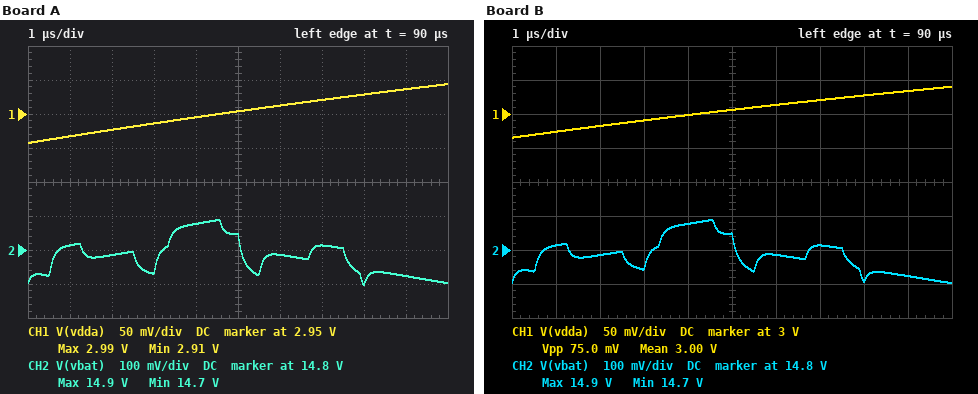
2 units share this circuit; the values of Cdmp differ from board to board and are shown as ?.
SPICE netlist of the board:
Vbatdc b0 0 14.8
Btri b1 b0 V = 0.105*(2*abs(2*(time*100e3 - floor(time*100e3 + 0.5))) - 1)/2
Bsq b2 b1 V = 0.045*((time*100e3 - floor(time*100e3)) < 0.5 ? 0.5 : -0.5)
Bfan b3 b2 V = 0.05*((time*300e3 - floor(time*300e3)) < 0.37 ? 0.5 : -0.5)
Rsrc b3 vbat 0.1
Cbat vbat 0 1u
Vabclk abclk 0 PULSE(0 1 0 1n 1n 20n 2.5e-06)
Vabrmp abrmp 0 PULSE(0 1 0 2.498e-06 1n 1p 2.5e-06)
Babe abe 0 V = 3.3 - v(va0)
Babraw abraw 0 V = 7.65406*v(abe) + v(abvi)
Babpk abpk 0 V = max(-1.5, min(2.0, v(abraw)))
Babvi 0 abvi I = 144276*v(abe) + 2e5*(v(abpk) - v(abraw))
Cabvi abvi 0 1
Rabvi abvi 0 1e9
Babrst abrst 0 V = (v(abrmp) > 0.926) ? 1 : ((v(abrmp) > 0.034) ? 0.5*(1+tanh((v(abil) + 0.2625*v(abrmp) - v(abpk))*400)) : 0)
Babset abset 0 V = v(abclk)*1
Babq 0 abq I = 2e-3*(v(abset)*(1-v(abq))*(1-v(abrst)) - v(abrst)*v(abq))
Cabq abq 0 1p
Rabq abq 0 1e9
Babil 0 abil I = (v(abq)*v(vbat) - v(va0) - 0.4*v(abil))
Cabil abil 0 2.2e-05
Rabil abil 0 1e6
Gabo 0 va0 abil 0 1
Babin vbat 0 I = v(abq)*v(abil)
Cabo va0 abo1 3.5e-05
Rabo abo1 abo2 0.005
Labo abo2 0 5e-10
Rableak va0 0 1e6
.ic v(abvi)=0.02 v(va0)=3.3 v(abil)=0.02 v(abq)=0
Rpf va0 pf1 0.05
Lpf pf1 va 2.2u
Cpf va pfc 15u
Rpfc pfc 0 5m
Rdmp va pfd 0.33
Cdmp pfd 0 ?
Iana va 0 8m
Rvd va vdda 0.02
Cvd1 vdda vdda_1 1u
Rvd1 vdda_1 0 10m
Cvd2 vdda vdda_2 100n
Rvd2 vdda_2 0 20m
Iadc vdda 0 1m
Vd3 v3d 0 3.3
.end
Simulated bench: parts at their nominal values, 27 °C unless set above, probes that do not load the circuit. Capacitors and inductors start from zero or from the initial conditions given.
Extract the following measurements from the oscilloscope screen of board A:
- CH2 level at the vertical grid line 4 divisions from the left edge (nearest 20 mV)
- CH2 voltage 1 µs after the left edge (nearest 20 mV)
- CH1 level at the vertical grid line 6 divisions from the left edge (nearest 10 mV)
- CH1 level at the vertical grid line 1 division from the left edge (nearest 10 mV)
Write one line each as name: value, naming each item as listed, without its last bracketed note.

CH2 level at the vertical grid line 4 divisions from the left edge: 14.88 V
CH2 voltage 1 µs after the left edge: 14.82 V
CH1 level at the vertical grid line 6 divisions from the left edge: 2.96 V
CH1 level at the vertical grid line 1 division from the left edge: 2.92 V
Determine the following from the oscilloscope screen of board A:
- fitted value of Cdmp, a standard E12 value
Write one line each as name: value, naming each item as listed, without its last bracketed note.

fitted value of Cdmp, a standard E12 value: 22 µF
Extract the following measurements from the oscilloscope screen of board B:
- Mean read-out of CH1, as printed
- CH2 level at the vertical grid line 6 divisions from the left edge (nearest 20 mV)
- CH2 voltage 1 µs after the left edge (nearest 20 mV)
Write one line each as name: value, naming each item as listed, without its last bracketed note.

Mean read-out of CH1, as printed: 3.00 V
CH2 level at the vertical grid line 6 divisions from the left edge: 14.78 V
CH2 voltage 1 µs after the left edge: 14.82 V
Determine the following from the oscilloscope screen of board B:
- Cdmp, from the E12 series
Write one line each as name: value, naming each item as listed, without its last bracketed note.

Cdmp, from the E12 series: 18 µF
